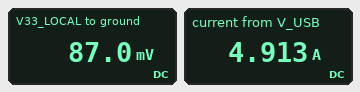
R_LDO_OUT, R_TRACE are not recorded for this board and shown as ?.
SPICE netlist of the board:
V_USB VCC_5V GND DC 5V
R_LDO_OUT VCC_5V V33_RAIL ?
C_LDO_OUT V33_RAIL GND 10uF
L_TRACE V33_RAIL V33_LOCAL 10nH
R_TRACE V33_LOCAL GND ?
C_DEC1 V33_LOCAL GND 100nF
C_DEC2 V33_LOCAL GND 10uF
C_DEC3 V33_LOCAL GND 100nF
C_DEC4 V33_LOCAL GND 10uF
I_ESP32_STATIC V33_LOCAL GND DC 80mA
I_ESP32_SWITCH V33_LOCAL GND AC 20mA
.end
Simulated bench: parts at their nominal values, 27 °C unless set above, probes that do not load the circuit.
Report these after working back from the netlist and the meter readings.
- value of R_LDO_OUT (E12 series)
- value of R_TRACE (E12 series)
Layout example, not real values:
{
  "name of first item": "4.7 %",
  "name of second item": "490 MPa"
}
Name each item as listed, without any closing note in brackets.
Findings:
{
  "value of R_LDO_OUT": "1 Ω",
  "value of R_TRACE": "0.018 Ω"
}
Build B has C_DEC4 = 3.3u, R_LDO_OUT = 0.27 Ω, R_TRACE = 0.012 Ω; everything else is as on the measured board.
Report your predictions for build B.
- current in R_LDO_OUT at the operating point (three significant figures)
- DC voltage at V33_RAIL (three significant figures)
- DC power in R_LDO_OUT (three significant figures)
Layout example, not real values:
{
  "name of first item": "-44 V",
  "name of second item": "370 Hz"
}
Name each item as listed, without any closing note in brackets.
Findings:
{
  "current in R_LDO_OUT at the operating point": "17.7 A",
  "DC voltage at V33_RAIL": "212 mV",
  "DC power in R_LDO_OUT": "84.9 W"
}
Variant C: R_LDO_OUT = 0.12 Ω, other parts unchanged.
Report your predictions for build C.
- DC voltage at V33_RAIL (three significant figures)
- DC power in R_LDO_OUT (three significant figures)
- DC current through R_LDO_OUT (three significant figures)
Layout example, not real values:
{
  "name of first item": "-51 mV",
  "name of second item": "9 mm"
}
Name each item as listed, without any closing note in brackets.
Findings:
{
  "DC voltage at V33_RAIL": "651 mV",
  "DC power in R_LDO_OUT": "158 W",
  "DC current through R_LDO_OUT": "36.2 A"
}
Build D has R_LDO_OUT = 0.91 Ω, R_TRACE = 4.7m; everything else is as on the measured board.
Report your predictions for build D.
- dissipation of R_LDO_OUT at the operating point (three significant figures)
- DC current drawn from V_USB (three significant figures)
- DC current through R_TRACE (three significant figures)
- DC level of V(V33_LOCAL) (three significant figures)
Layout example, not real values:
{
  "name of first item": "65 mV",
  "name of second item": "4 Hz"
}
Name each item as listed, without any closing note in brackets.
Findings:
{
  "dissipation of R_LDO_OUT at the operating point": "27.2 W",
  "DC current drawn from V_USB": "5.47 A",
  "DC current through R_TRACE": "5.39 A",
  "DC level of V(V33_LOCAL)": "25.3 mV"
}
